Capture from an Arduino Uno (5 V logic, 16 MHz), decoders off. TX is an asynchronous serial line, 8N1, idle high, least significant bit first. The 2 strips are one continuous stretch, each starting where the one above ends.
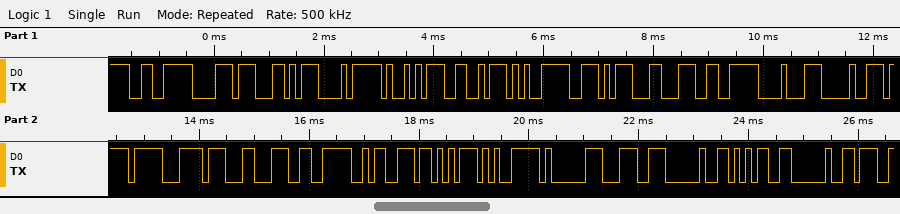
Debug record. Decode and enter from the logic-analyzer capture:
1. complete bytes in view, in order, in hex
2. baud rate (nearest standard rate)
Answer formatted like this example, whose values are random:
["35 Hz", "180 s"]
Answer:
["E6 B8 AC E8 A9 A6 E5 AE 8C E6 88 90 EF BC 8C E6 9A AB E5 81 9C 20 35 20", "9600 baud"]
